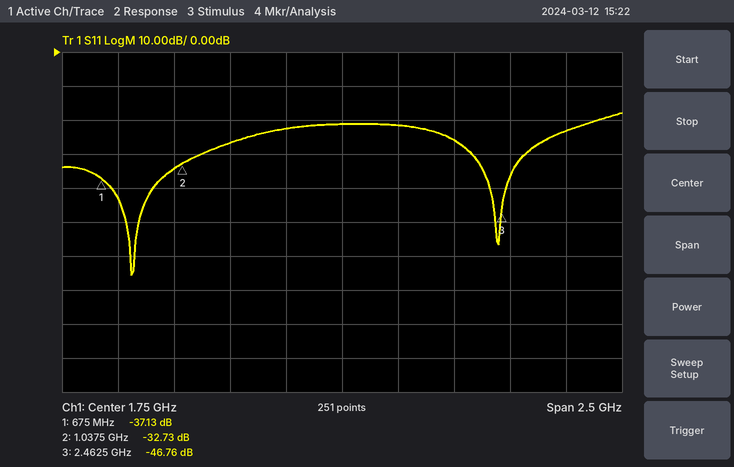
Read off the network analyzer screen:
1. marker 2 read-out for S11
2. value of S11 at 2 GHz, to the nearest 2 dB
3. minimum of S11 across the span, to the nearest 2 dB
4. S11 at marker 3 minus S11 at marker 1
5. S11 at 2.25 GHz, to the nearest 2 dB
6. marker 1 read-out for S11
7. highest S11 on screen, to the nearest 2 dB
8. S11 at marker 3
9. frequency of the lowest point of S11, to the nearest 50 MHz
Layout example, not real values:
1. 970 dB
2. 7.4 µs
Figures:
1. -32.73 dB
2. -22 dB
3. -66 dB
4. -9.63 dB
5. -26 dB
6. -37.13 dB
7. -18 dB
8. -46.76 dB
9. 800 MHz
